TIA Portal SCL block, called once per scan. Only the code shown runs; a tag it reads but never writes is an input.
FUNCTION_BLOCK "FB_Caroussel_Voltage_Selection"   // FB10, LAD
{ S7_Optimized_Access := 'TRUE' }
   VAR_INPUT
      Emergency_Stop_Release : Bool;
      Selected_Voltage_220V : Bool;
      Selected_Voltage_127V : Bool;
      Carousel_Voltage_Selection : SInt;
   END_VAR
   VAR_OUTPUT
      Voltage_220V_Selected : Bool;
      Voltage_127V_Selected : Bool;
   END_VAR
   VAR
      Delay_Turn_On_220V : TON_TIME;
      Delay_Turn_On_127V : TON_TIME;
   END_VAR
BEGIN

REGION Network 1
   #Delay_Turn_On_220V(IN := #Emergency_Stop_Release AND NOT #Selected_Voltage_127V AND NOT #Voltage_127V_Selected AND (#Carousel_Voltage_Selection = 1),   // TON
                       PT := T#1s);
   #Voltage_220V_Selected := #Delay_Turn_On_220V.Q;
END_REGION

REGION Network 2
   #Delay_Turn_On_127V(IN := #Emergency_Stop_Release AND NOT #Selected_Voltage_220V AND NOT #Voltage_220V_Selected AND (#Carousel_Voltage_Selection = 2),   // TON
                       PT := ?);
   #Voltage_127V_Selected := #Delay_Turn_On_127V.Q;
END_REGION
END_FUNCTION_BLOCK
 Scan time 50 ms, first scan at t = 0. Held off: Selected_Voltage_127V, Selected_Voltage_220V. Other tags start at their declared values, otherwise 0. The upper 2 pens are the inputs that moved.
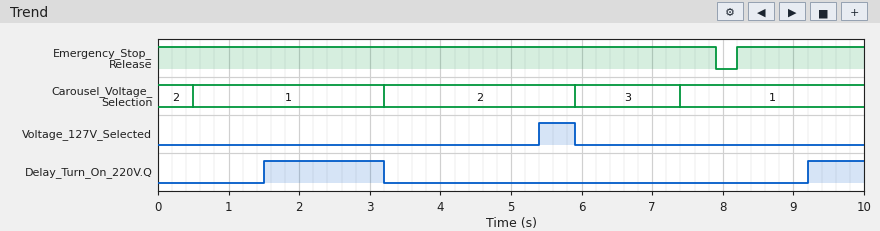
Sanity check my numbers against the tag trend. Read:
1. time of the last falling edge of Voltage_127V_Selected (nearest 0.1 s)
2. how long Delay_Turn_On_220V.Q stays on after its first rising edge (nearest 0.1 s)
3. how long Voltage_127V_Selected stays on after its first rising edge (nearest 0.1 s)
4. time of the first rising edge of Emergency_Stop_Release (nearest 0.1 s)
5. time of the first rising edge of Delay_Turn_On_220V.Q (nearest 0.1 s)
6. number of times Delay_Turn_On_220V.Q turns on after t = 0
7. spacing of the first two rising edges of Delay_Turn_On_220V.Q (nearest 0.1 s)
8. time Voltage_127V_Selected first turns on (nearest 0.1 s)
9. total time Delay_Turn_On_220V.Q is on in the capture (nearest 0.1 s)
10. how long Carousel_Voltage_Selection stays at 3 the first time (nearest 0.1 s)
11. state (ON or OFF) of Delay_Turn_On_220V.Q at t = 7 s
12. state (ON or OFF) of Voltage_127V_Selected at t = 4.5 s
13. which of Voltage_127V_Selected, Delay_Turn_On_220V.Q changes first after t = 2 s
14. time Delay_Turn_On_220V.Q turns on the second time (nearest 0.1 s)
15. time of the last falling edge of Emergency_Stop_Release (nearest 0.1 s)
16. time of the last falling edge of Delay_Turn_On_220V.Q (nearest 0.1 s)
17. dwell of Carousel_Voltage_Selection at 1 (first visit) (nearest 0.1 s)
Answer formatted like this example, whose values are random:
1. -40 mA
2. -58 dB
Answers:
1. 5.9 s
2. 1.7 s
3. 0.5 s
4. 8.2 s
5. 1.5 s
6. 2
7. 7.7 s
8. 5.4 s
9. 2.5 s
10. 1.5 s
11. OFF
12. OFF
13. Delay_Turn_On_220V.Q
14. 9.2 s
15. 7.9 s
16. 3.2 s
17. 2.7 s
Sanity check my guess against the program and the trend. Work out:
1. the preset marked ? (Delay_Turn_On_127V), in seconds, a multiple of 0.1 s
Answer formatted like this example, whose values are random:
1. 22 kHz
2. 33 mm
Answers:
1. 2.2 s
